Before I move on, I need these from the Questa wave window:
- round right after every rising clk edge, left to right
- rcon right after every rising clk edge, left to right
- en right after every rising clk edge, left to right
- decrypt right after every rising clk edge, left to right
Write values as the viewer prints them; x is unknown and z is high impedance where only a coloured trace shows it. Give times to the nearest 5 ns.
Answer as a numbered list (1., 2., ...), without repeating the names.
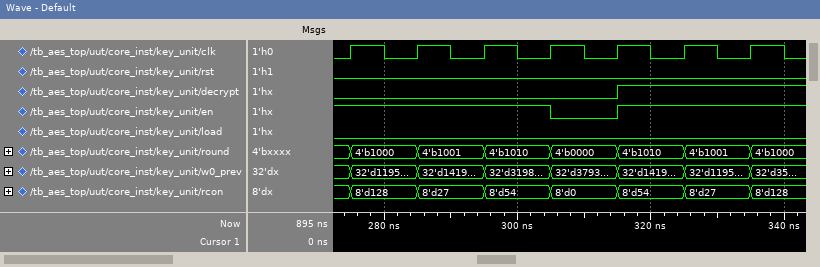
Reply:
1. 4'b1000, 4'b1001, 4'b1010, 4'b0000, 4'b1010, 4'b1001, 4'b1000
2. 8'd128, 8'd27, 8'd54, 8'd0, 8'd54, 8'd27, 8'd128
3. 1 1 1 0 1 1 1
4. 0 0 0 0 1 1 1
